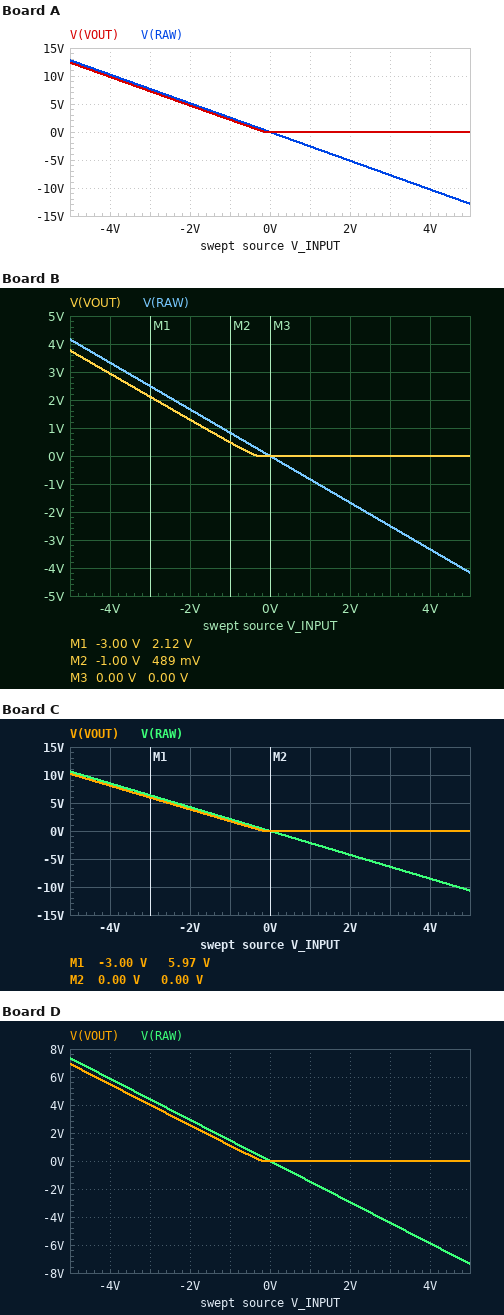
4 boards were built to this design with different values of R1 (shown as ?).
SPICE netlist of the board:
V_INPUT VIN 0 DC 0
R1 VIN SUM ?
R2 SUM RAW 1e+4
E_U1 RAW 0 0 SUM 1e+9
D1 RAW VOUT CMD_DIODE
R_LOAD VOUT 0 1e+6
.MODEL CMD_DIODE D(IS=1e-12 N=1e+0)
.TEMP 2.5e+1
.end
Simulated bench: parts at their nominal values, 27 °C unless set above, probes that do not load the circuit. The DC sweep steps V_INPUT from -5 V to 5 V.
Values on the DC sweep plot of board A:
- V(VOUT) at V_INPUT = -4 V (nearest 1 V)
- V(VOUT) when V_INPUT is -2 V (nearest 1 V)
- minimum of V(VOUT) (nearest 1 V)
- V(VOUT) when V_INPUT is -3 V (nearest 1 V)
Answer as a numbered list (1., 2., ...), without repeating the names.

1. 10 V
2. 5 V
3. 0 V
4. 7 V
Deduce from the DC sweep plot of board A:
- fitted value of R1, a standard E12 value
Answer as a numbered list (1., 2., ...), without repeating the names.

1. 3.9 kΩ
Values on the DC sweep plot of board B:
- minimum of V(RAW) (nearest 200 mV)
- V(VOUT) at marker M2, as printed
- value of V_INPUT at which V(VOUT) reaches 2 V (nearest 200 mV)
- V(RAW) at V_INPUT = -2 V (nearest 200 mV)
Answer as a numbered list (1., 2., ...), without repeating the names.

1. -4.2 V
2. 489 mV
3. -2.8 V
4. 1.6 V
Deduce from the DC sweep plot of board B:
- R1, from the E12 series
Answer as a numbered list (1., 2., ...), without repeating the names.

1. 12 kΩ
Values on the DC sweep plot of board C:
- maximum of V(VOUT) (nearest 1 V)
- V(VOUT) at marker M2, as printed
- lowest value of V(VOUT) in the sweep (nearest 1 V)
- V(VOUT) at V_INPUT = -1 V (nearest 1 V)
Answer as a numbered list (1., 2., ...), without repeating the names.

1. 10 V
2. 0.00 V
3. 0 V
4. 2 V
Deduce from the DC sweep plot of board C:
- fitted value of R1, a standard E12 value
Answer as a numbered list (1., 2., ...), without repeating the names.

1. 4.7 kΩ
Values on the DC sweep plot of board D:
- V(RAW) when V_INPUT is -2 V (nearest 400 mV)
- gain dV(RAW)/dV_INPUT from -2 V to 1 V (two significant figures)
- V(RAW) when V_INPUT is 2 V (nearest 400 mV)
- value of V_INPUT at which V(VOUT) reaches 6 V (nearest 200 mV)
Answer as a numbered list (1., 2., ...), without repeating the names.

1. 2.8 V
2. -1.5 V/V
3. -2.8 V
4. -4.4 V
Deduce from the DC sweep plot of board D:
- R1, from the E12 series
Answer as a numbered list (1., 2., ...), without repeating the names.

1. 6.8 kΩ
